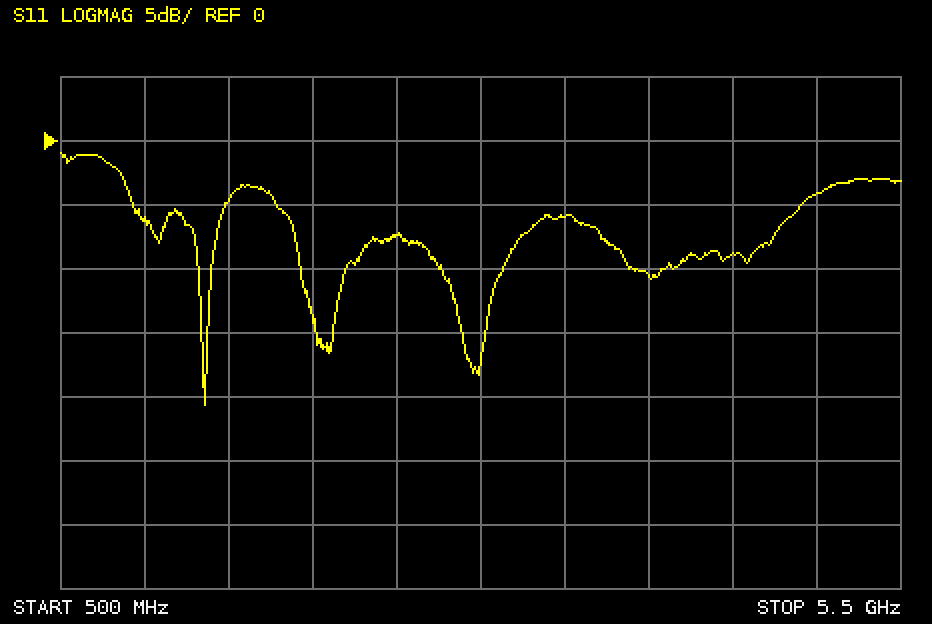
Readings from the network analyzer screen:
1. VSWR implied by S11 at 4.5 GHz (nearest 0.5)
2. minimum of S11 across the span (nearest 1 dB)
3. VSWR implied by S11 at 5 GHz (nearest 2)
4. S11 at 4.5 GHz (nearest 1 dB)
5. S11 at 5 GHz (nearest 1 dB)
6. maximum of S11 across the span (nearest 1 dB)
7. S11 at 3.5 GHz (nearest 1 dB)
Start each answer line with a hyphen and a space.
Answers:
- 2.0
- -21 dB
- 4
- -9 dB
- -4 dB
- -1 dB
- -6 dB
